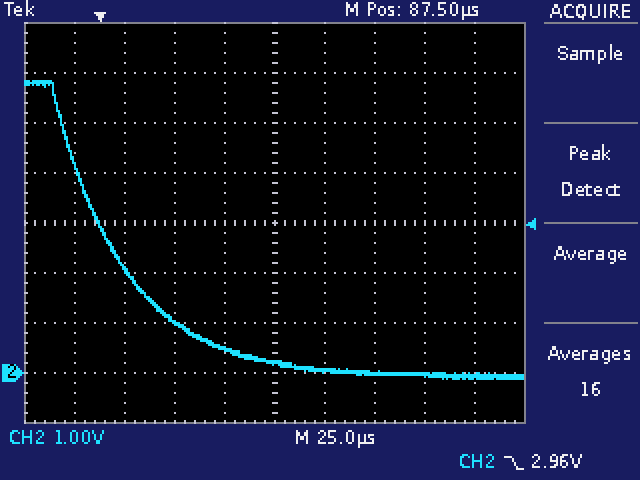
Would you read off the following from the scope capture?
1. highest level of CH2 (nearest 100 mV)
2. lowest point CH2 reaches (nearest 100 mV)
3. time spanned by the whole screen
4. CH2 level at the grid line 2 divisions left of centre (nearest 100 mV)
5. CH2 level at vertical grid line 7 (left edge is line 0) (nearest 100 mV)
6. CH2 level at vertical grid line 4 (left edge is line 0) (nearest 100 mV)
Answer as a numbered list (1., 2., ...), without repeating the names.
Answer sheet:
1. 5.8 V
2. -100 mV
3. 250 µs
4. 1.0 V
5. 0.0 V
6. 500 mV
